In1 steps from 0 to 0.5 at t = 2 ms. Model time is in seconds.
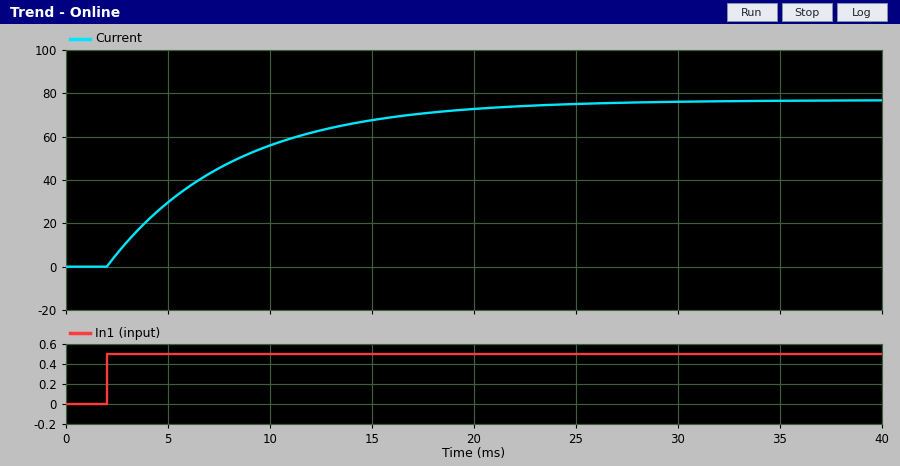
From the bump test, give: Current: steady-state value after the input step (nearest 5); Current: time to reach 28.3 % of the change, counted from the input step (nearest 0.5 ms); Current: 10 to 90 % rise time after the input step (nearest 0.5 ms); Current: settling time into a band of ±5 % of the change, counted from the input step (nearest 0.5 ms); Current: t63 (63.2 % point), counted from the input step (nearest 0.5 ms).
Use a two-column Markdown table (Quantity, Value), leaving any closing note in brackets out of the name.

| Quantity | Value |
|---|---|
| Current: steady-state value after the input step | 75 |
| Current: time to reach 28.3 % of the change, counted from the input step | 2.0 ms |
| Current: 10 to 90 % rise time after the input step | 13.5 ms |
| Current: settling time into a band of ±5 % of the change, counted from the input step | 18.5 ms |
| Current: t63 (63.2 % point), counted from the input step | 6.0 ms |
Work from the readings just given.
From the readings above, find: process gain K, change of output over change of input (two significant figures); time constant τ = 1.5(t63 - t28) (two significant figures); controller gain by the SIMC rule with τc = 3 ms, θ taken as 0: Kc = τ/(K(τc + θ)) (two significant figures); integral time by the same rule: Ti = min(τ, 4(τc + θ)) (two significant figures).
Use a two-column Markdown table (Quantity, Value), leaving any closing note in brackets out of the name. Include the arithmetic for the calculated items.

| Quantity | Value |
|---|---|
| process gain K, change of output over change of input | (75 - 0) / 0.5 = 150 |
| time constant τ = 1.5(t63 - t28) | 1.5 × (6 - 2) = 6.0 ms |
| controller gain by the SIMC rule with τc = 3 ms, θ taken as 0: Kc = τ/(K(τc + θ)) | 6 / (150 × (3 + 0)) = 0.013 |
| integral time by the same rule: Ti = min(τ, 4(τc + θ)) | min(6, 4 × (3 + 0)) = 6.0 ms |
